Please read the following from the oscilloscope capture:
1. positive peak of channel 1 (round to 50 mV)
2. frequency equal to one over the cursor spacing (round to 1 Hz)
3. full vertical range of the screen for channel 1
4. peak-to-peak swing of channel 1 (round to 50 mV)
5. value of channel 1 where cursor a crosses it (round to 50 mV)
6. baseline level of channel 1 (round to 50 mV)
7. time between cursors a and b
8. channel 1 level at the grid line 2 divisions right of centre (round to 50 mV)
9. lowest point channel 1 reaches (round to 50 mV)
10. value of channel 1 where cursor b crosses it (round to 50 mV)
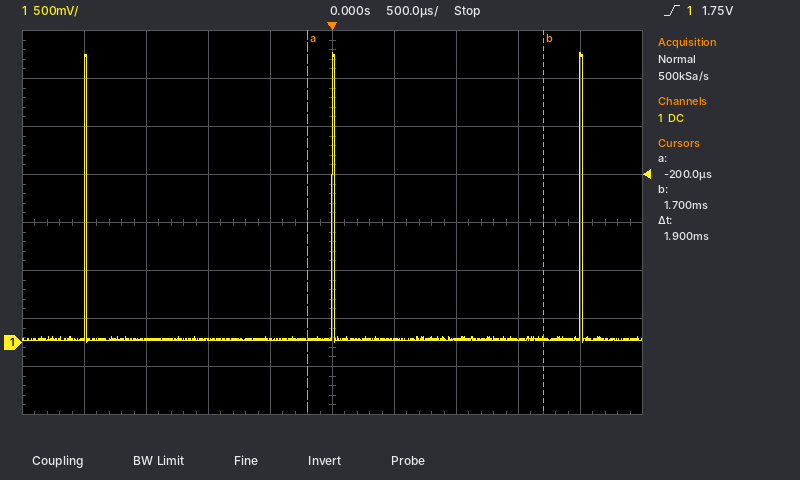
3.00 V
526 Hz
4 V
3.00 V
50 mV
50 mV
1.9 ms
50 mV
0 mV
50 mV
